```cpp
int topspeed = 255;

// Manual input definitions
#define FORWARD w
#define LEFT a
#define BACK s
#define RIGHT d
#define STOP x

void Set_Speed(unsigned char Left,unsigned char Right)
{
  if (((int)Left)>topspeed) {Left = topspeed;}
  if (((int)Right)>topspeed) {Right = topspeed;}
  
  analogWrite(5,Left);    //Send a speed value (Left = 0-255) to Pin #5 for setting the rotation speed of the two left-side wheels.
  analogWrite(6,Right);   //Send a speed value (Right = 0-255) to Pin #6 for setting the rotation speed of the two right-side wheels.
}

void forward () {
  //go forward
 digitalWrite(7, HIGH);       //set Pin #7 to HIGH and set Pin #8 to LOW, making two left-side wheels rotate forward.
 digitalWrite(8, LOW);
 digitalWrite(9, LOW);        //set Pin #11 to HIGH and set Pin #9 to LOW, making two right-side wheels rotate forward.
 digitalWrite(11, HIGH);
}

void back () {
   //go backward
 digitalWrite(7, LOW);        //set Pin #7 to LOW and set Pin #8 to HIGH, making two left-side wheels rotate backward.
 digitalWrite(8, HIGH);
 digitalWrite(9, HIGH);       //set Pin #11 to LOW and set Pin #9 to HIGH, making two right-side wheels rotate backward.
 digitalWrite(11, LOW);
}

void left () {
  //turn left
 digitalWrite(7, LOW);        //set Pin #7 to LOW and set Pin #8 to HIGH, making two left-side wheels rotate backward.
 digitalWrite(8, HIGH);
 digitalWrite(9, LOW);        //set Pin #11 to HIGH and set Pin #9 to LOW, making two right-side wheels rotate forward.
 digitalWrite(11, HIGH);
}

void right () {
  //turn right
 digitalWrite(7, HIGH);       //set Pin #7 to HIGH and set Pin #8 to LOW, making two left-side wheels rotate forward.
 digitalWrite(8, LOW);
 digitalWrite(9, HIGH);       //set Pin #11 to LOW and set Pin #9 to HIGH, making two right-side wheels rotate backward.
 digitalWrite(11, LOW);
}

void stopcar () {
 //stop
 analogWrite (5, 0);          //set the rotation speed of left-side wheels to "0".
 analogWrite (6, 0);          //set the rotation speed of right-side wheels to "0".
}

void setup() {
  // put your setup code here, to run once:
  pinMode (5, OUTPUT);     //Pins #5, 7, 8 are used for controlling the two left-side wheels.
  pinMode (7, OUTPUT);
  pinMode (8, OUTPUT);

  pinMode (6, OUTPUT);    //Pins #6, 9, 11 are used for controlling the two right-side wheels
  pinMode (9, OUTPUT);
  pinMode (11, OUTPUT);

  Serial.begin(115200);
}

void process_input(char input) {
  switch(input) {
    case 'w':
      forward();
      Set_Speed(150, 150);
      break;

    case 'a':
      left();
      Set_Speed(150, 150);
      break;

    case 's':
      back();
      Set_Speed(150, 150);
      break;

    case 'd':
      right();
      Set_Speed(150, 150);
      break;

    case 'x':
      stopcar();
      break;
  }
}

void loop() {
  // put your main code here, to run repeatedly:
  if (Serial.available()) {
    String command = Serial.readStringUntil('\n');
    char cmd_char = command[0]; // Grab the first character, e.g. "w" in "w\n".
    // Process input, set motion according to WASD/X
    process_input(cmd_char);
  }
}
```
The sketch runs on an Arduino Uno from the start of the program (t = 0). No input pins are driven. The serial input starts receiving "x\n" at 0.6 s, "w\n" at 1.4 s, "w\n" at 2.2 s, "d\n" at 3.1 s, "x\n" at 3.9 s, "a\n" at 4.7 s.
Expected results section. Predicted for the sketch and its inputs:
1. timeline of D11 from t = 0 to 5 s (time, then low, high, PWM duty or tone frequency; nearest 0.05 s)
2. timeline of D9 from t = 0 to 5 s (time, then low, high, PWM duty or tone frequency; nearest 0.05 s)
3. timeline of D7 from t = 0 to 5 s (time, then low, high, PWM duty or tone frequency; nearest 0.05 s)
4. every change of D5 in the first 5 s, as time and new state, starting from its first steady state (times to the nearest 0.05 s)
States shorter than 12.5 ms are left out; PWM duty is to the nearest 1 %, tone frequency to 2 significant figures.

0 s low; 1.4 s high; 3.1 s low; 4.7 s high
0 s low; 3.1 s high; 4.7 s low
0 s low; 1.4 s high; 4.7 s low
0 s low; 1.4 s PWM 59 %; 3.9 s low; 4.7 s PWM 59 %
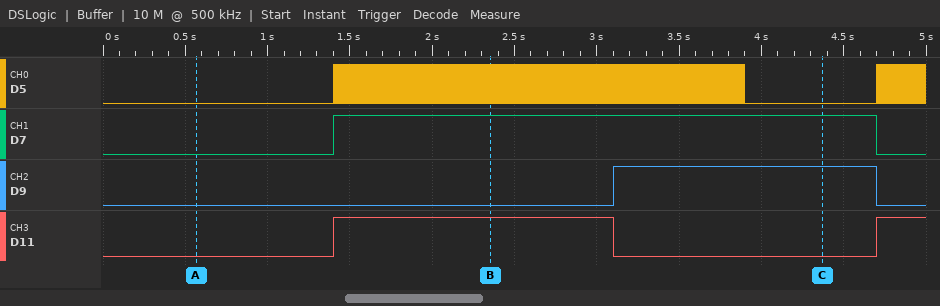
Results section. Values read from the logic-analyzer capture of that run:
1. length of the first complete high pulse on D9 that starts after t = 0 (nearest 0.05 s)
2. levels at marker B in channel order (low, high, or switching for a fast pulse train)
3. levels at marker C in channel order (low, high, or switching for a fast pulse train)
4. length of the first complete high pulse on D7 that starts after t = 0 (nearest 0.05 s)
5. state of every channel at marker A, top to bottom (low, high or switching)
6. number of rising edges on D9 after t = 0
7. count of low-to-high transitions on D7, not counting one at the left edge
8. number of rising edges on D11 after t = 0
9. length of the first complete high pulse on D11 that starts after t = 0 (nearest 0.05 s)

1.60 s
D5 switching, D7 high, D9 low, D11 high
D5 low, D7 high, D9 high, D11 low
3.30 s
D5 low, D7 low, D9 low, D11 low
1
1
2
1.70 s
